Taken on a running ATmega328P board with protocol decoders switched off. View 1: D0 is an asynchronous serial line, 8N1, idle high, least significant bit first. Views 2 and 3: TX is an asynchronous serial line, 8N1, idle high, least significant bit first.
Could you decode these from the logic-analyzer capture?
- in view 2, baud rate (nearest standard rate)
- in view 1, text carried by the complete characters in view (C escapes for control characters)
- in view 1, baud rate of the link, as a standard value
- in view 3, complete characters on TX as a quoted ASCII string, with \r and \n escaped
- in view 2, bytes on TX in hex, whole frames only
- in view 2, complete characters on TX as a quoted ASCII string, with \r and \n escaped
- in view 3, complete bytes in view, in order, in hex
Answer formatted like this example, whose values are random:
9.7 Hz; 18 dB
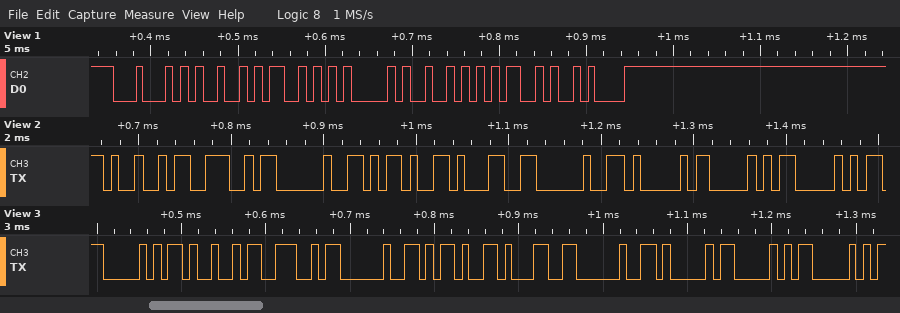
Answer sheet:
115200 baud; "DISARM\n"; 115200 baud; "PIN -1 APP"; 49 4E 20 2D 31 20 41 50 50; "IN -1 APP"; 50 49 4E 20 2D 31 20 41 50 50
